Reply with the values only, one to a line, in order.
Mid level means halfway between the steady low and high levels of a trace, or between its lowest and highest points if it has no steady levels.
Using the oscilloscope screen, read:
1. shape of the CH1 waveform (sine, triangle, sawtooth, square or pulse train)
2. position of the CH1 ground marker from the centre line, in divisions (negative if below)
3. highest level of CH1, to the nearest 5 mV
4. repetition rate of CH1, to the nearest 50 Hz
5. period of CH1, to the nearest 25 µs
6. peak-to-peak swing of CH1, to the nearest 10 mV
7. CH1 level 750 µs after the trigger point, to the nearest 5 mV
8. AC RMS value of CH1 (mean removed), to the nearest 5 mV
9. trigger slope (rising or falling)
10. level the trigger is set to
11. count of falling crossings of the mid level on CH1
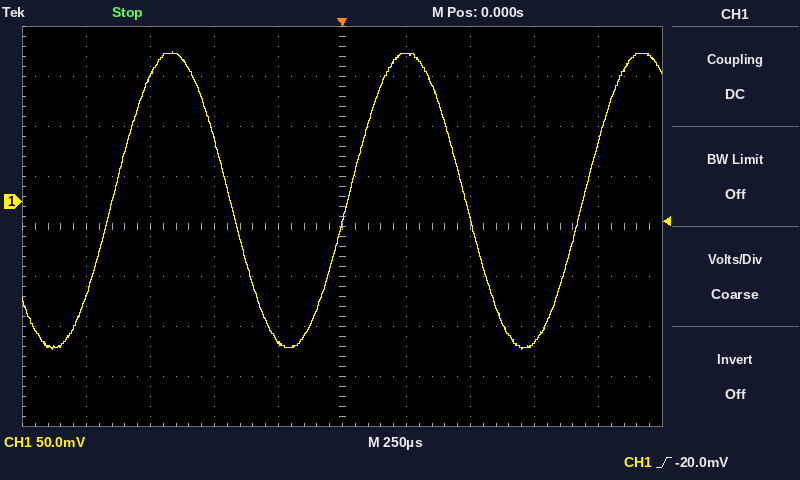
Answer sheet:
sine
+0.5 div
150 mV
1.10 kHz
925 µs
300 mV
-140 mV
105 mV
rising
-20.0 mV
2
